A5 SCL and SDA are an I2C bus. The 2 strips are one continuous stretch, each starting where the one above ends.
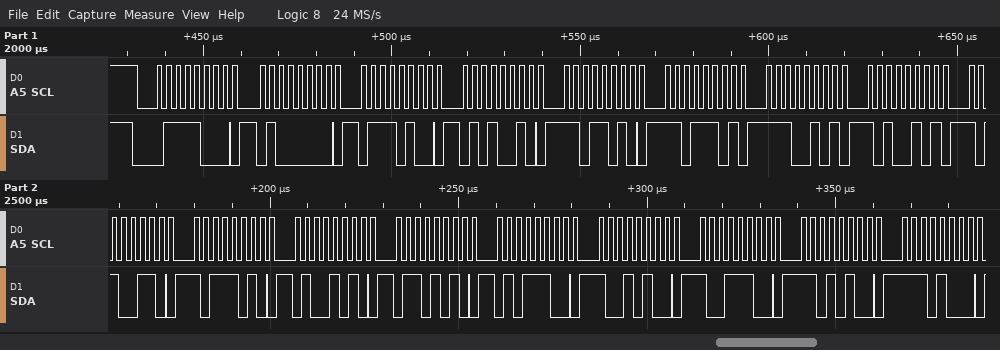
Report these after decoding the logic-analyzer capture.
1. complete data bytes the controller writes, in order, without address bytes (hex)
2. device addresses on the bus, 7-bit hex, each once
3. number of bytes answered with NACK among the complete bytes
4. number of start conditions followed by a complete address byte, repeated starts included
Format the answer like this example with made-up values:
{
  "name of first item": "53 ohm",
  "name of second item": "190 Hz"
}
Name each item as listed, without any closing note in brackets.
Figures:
{
  "complete data bytes the controller writes, in order, without address bytes": "40 74 52 DA DD E5 A5 A6 BA 4A 6A 5C 94 9C D4 E8",
  "device addresses on the bus, 7-bit hex, each once": "0x3C",
  "number of bytes answered with NACK among the complete bytes": "0",
  "number of start conditions followed by a complete address byte, repeated starts included": "1"
}
